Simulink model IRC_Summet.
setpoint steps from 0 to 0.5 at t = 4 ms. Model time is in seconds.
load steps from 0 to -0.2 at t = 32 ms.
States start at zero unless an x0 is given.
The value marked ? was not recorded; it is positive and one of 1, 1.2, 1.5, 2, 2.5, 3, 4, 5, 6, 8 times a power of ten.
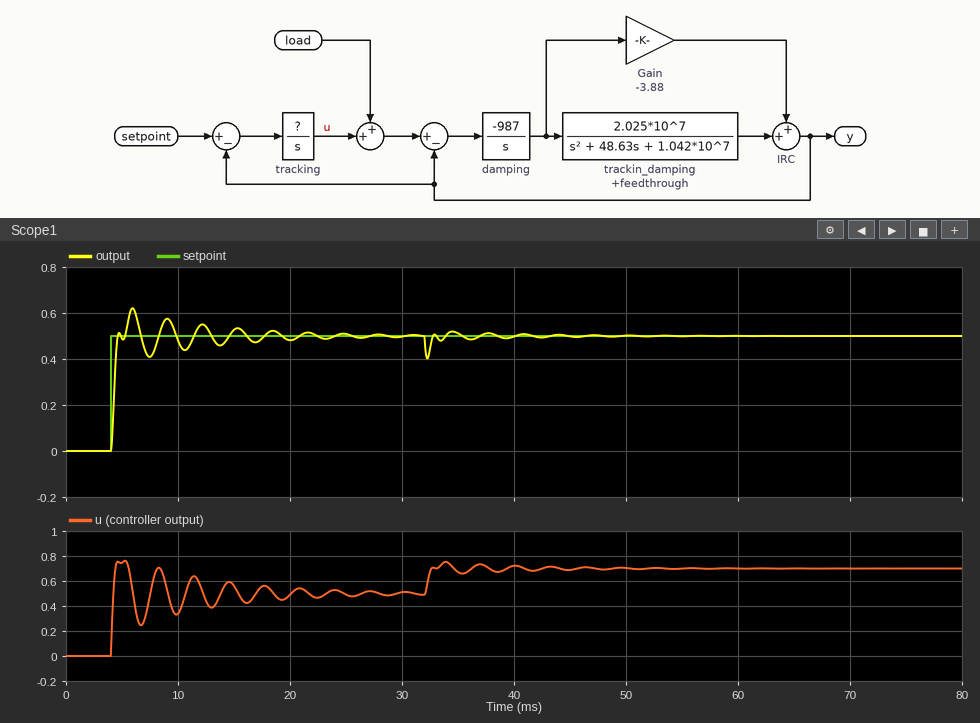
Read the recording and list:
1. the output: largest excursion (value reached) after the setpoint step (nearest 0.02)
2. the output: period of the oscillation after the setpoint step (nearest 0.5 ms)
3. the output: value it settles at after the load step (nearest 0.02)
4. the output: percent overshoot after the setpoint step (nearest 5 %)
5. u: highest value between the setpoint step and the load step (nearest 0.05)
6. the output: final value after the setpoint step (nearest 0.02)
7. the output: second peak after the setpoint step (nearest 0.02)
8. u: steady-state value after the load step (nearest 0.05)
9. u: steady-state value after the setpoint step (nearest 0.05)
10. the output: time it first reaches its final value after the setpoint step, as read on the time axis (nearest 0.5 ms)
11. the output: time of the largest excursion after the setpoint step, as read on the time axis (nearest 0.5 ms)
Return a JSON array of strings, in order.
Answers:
["0.62", "3.0 ms", "0.50", "25 %", "0.75", "0.50", "0.58", "0.70", "0.50", "4.5 ms", "6.0 ms"]
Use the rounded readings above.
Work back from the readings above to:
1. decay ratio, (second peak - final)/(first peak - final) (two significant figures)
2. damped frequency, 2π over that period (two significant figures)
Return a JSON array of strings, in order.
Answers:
["0.67", "2.1 rad/ms"]
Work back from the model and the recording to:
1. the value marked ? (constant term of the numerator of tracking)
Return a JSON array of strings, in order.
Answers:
["5000"]
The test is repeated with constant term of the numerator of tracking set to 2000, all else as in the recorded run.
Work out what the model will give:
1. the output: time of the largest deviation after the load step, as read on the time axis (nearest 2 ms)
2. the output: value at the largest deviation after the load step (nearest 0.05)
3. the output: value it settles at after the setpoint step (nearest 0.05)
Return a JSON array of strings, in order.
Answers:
["32 ms", "0.40", "0.50"]
